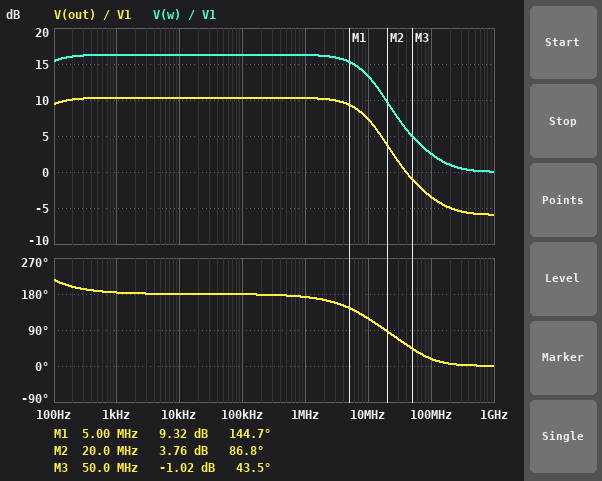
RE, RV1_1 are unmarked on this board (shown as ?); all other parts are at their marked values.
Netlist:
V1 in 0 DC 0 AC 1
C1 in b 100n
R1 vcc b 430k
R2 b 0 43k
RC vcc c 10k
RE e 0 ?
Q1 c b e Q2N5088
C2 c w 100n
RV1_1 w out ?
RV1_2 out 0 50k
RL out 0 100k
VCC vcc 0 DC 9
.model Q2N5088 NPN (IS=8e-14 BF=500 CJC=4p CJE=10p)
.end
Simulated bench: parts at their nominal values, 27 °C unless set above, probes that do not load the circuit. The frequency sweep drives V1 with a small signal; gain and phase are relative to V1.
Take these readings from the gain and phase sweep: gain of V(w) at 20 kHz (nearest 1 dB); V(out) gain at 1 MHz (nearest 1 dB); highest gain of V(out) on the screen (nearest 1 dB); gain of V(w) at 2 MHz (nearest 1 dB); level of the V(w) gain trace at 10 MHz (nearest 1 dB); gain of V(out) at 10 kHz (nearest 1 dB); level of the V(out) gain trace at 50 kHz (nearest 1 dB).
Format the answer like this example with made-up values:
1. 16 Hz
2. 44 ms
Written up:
1. 16 dB
2. 10 dB
3. 10 dB
4. 16 dB
5. 13 dB
6. 10 dB
7. 10 dB
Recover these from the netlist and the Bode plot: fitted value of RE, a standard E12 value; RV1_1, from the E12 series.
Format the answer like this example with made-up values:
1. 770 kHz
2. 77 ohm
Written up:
1. 1.2 kΩ
2. 33 kΩ
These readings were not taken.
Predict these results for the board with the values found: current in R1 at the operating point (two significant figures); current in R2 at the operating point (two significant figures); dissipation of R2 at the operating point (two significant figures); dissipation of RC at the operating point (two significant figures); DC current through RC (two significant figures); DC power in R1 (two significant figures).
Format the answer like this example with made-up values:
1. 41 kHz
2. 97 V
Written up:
1. 19 µA
2. 19 µA
3. 15 µW
4. 410 µW
5. 200 µA
6. 160 µW
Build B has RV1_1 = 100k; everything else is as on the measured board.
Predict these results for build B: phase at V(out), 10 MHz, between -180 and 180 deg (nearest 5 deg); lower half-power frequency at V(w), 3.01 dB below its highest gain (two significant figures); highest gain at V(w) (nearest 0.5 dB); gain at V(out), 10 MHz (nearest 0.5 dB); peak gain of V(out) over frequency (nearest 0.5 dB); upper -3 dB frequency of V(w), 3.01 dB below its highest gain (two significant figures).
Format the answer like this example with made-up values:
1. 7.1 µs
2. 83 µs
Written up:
1. 115 deg
2. 46 Hz
3. 17.0 dB
4. 1.5 dB
5. 5.0 dB
6. 9.3 MHz
